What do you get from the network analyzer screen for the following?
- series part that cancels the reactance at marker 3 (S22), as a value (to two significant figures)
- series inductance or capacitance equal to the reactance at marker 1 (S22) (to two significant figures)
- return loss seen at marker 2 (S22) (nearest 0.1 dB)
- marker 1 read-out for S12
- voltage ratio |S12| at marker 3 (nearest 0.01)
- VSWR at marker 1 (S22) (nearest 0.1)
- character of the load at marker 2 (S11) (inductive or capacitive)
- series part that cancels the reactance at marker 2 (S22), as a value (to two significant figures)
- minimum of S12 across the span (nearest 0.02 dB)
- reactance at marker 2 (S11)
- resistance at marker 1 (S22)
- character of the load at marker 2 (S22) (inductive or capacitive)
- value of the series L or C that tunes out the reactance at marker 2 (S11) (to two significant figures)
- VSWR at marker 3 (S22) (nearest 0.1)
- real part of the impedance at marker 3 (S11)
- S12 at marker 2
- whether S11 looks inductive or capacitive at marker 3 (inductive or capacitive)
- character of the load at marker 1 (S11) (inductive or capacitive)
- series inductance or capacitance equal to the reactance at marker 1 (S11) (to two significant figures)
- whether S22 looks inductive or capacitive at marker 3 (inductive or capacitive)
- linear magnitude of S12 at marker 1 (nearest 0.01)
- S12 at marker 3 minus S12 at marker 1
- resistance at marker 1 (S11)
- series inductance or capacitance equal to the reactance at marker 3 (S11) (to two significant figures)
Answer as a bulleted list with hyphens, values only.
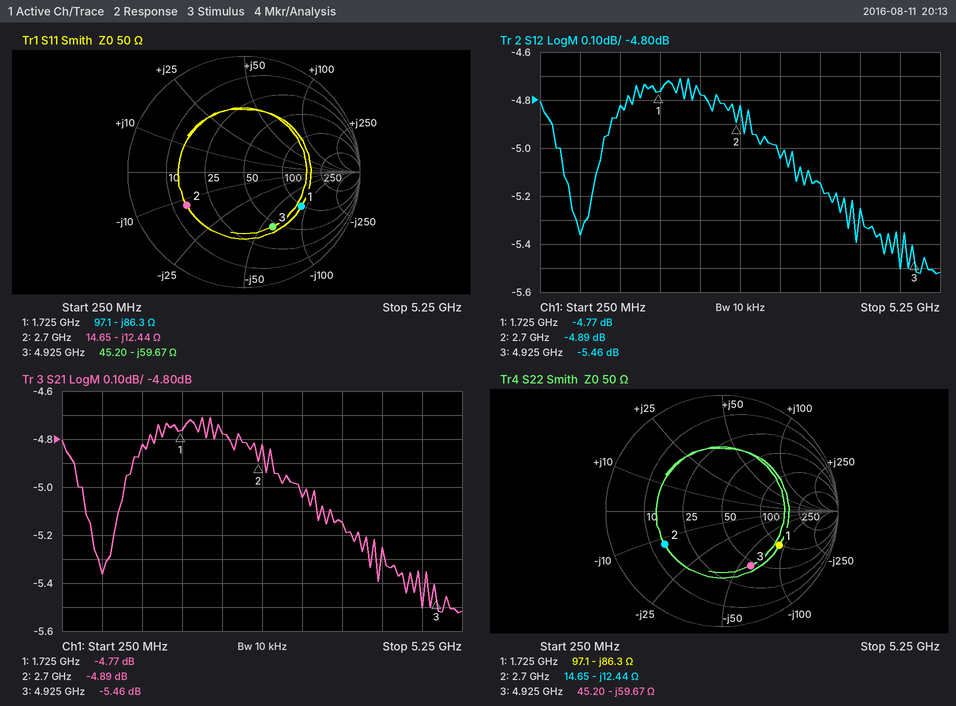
- 1.9 nH
- 1.1 pF
- 4.9 dB
- -4.77 dB
- 0.53
- 3.7
- capacitive
- 730 pH
- -5.52 dB
- -12.44 Ω
- 97.1 Ω
- capacitive
- 730 pH
- 3.3
- 45.20 Ω
- -4.89 dB
- capacitive
- capacitive
- 1.1 pF
- capacitive
- 0.58
- -0.69 dB
- 97.1 Ω
- 540 fF
